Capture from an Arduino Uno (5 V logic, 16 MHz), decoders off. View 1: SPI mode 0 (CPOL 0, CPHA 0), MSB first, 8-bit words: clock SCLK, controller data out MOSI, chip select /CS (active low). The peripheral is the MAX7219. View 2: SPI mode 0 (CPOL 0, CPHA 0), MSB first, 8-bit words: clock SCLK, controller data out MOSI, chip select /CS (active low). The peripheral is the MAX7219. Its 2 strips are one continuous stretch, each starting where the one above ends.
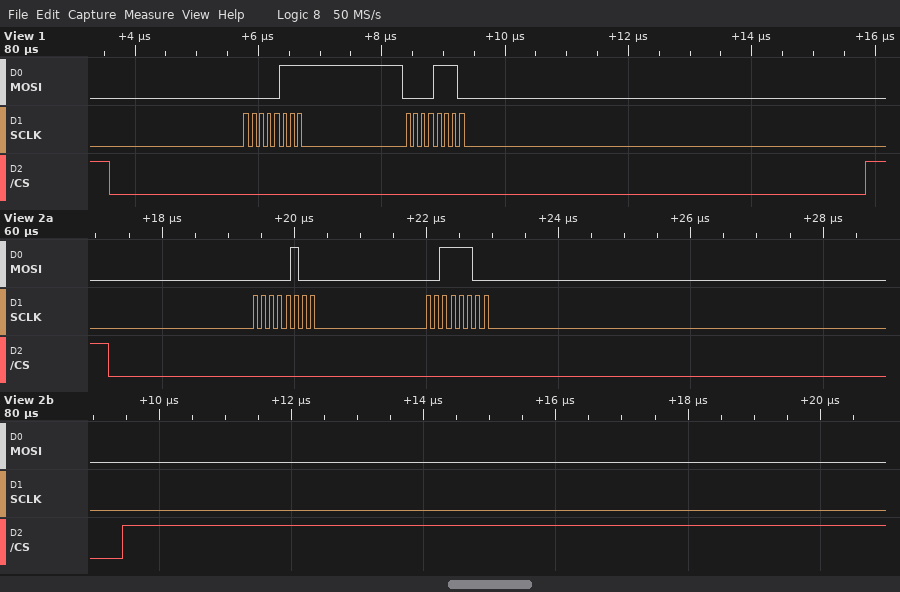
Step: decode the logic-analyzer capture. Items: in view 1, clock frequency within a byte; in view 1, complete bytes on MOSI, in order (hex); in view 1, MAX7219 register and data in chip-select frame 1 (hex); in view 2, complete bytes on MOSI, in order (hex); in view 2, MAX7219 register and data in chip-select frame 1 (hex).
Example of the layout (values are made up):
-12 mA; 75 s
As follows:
8 MHz; 07 0E; register 0x7, data 0x0E; 04 3C; register 0x4, data 0x3C
